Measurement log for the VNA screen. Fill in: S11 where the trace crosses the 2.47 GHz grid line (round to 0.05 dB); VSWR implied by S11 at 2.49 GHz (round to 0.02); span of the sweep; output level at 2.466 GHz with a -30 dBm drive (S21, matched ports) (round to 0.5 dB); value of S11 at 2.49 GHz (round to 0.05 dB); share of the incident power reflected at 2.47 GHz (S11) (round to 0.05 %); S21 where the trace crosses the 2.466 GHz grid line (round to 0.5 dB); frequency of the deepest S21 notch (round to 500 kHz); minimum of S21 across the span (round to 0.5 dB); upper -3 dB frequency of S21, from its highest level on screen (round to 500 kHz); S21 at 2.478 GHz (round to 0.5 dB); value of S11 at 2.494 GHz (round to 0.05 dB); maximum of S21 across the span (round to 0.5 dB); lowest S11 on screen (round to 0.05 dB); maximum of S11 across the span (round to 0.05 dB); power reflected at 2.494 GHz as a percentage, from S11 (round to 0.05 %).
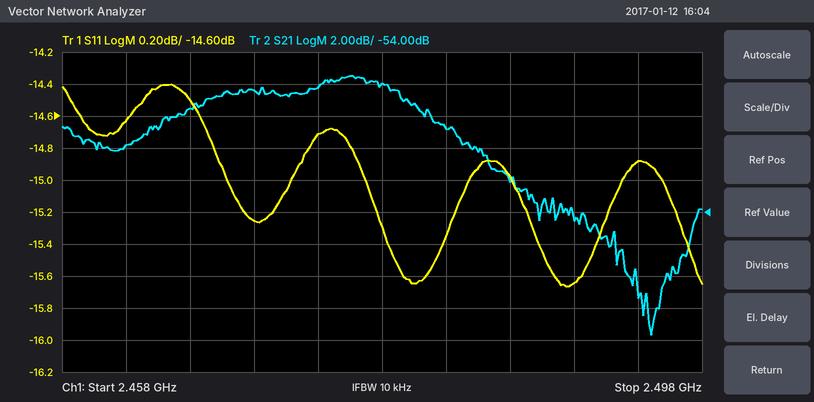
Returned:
-15.25 dB
1.40
40 MHz
-77.5 dBm
-15.65 dB
3.00 %
-47.5 dB
2.4950 GHz
-61.5 dB
2.4815 GHz
-46.0 dB
-14.90 dB
-45.5 dB
-15.65 dB
-14.40 dB
3.25 %
